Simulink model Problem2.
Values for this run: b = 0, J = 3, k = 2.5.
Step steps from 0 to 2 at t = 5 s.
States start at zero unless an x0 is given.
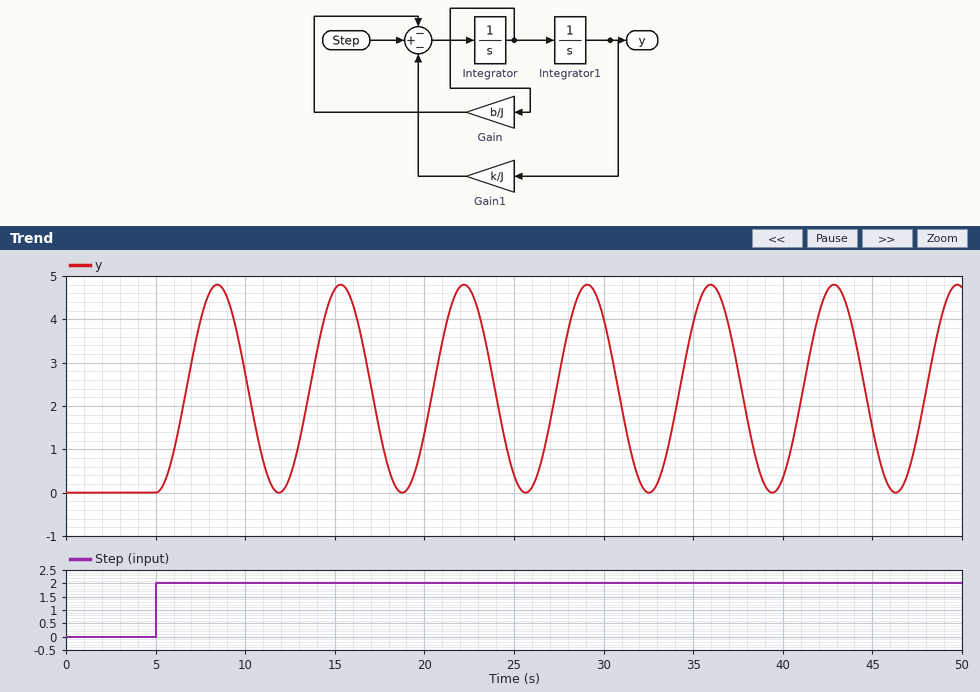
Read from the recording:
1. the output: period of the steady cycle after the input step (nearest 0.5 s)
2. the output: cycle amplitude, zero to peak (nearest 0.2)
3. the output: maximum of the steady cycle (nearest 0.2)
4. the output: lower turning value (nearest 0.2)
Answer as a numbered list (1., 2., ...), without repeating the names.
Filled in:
1. 7.0 s
2. 2.4
3. 4.8
4. 0.0
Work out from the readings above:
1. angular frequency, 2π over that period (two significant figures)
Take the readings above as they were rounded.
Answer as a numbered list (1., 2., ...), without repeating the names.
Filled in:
1. 0.90 rad/s
